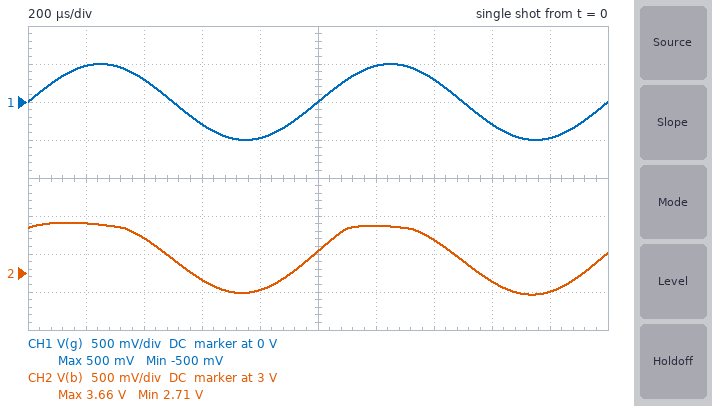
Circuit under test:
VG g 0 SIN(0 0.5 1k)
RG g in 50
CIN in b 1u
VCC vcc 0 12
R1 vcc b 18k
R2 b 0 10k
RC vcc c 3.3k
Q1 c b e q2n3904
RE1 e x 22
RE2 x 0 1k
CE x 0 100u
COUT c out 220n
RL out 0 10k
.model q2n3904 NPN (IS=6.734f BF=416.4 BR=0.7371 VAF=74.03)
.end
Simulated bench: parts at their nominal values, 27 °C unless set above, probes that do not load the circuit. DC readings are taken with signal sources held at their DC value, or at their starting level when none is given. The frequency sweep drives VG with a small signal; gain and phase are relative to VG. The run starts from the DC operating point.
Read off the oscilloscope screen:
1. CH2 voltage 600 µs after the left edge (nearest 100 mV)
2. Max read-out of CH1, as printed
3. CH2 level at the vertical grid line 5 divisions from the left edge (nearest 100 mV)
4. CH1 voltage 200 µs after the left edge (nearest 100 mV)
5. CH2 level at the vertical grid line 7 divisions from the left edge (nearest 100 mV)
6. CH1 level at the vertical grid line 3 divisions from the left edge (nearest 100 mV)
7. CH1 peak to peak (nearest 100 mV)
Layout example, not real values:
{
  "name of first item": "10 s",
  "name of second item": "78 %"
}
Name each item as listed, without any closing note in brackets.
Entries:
{
  "CH2 voltage 600 µs after the left edge": "2.9 V",
  "Max read-out of CH1, as printed": "500 mV",
  "CH2 level at the vertical grid line 5 divisions from the left edge": "3.3 V",
  "CH1 voltage 200 µs after the left edge": "500 mV",
  "CH2 level at the vertical grid line 7 divisions from the left edge": "3.4 V",
  "CH1 level at the vertical grid line 3 divisions from the left edge": "-300 mV",
  "CH1 peak to peak": "1.0 V"
}
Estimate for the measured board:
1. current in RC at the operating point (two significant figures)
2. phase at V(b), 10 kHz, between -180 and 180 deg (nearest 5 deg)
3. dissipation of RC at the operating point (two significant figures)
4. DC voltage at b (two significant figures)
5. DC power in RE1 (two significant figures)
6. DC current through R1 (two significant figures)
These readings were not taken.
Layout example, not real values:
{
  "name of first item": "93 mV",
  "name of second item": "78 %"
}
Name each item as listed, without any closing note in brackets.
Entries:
{
  "current in RC at the operating point": "2.7 mA",
  "phase at V(b), 10 kHz, between -180 and 180 deg": "10 deg",
  "dissipation of RC at the operating point": "25 mW",
  "DC voltage at b": "3.6 V",
  "DC power in RE1": "180 µW",
  "DC current through R1": "470 µA"
}
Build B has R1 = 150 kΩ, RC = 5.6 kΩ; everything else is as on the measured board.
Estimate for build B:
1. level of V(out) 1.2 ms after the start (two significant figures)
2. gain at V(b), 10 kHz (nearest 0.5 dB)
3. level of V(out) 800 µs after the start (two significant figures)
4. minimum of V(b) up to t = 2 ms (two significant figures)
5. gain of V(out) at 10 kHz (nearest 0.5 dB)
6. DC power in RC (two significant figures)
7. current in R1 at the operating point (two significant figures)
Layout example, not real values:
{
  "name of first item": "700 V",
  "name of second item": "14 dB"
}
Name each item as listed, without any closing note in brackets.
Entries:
{
  "level of V(out) 1.2 ms after the start": "-9.6 V",
  "gain at V(b), 10 kHz": "0 dB",
  "level of V(out) 800 µs after the start": "1.3 V",
  "minimum of V(b) up to t = 2 ms": "-43 mV",
  "gain of V(out) at 10 kHz": "24.5 dB",
  "DC power in RC": "100 µW",
  "current in R1 at the operating point": "75 µA"
}
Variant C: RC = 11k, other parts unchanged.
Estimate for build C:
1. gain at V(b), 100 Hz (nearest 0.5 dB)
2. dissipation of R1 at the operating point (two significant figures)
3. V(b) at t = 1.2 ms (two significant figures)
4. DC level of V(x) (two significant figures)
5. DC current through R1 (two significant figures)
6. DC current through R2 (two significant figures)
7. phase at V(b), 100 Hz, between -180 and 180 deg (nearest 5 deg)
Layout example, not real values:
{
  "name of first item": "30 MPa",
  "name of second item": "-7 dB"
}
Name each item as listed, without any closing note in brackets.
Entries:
{
  "gain at V(b), 100 Hz": "-29.5 dB",
  "dissipation of R1 at the operating point": "5.5 mW",
  "V(b) at t = 1.2 ms": "2.1 V",
  "DC level of V(x)": "1.3 V",
  "DC current through R1": "550 µA",
  "DC current through R2": "200 µA",
  "phase at V(b), 100 Hz, between -180 and 180 deg": "70 deg"
}
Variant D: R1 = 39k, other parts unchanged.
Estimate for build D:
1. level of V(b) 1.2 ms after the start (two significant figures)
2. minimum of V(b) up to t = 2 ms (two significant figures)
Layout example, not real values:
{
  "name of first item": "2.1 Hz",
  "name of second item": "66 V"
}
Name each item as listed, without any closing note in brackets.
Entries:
{
  "level of V(b) 1.2 ms after the start": "2.5 V",
  "minimum of V(b) up to t = 2 ms": "1.5 V"
}
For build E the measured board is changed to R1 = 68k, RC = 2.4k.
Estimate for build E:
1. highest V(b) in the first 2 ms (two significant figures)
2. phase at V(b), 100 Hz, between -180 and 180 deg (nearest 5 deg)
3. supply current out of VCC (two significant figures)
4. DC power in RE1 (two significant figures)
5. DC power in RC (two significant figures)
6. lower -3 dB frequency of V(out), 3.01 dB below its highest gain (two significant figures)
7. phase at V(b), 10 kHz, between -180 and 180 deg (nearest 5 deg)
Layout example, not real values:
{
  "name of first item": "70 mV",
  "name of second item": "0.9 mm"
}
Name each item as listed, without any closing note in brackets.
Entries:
{
  "highest V(b) in the first 2 ms": "1.7 V",
  "phase at V(b), 100 Hz, between -180 and 180 deg": "15 deg",
  "supply current out of VCC": "1.0 mA",
  "DC power in RE1": "16 µW",
  "DC power in RC": "1.7 mW",
  "lower -3 dB frequency of V(out), 3.01 dB below its highest gain": "81 Hz",
  "phase at V(b), 10 kHz, between -180 and 180 deg": "0 deg"
}
